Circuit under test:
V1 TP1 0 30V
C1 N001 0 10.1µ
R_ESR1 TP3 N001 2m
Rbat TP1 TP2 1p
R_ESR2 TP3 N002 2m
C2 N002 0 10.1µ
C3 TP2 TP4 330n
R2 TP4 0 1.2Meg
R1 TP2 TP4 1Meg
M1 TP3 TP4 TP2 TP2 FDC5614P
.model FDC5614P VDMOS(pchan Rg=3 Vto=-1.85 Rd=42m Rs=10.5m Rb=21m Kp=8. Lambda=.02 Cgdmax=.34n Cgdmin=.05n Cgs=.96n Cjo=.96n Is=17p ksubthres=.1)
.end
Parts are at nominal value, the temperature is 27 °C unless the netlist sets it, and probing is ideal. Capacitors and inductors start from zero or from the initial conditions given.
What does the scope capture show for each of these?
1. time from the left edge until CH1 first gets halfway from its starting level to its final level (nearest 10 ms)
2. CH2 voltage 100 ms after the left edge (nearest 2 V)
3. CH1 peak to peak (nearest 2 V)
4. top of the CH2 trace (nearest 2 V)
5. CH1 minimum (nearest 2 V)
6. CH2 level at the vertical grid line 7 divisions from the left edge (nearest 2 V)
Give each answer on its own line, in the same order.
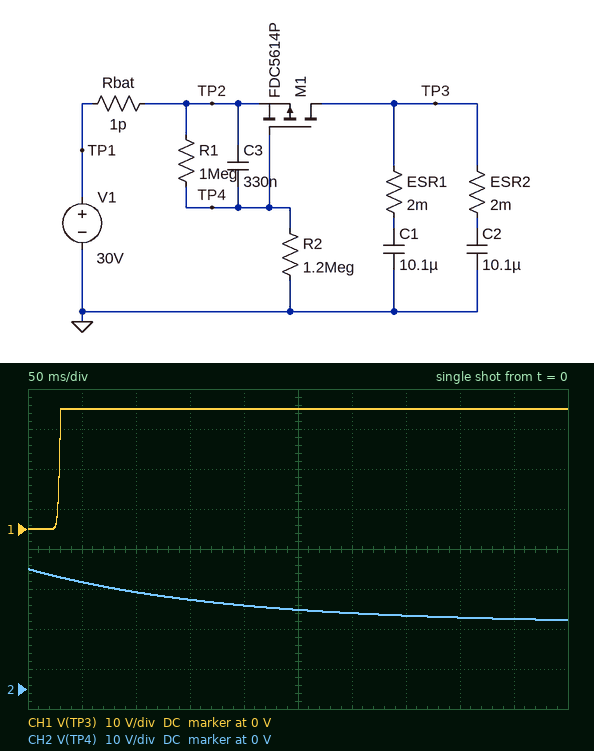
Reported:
30 ms
24 V
30 V
30 V
0 V
18 V
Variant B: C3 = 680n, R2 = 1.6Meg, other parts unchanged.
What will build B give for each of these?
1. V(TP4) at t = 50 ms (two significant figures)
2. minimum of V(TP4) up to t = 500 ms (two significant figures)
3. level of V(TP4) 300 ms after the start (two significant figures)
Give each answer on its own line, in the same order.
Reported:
29 V
22 V
24 V
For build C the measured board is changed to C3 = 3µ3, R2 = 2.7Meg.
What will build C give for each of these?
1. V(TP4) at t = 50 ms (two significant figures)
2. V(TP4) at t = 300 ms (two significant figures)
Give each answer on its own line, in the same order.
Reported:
30 V
29 V
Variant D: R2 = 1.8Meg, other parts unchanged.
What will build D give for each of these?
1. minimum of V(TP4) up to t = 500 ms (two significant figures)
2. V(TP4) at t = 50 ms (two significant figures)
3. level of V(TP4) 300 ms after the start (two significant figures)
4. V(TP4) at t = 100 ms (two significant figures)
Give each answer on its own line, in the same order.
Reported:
20 V
28 V
22 V
26 V
